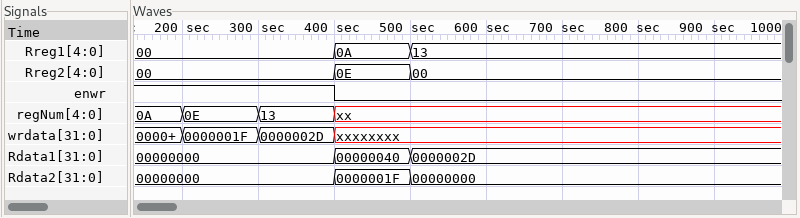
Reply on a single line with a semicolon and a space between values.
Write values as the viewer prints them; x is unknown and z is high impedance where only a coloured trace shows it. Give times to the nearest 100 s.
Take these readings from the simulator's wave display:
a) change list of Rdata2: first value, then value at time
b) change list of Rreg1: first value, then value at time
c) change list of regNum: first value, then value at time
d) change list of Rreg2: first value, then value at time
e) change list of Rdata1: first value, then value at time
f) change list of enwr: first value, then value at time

00000000, 0000001F at 400 s, 00000000 at 500 s; 00, 0A at 400 s, 13 at 500 s; 0A, 0E at 200 s, 13 at 300 s, xx at 400 s; 00, 0E at 400 s, 00 at 500 s; 00000000, 00000040 at 400 s, 0000002D at 500 s; 1, 0 at 400 s
